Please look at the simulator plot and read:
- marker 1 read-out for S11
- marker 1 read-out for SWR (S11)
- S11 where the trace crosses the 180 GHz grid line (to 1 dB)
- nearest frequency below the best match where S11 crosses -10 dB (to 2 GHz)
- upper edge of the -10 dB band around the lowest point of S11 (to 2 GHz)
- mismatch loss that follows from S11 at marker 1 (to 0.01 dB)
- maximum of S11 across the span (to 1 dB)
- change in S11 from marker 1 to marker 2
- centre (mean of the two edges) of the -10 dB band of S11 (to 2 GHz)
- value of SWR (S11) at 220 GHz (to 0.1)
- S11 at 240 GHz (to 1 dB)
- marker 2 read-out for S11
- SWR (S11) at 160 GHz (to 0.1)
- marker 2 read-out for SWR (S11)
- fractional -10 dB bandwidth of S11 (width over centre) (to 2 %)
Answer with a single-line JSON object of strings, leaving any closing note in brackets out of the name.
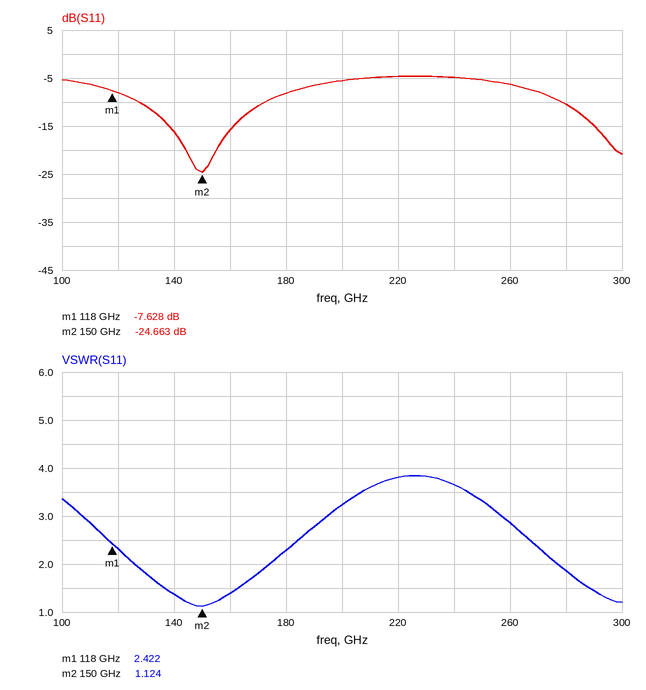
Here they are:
{"marker 1 read-out for S11": "-7.628 dB", "marker 1 read-out for SWR": "2.422", "S11 where the trace crosses the 180 GHz grid line": "-8 dB", "nearest frequency below the best match where S11 crosses -10 dB": "128 GHz", "upper edge of the -10 dB band around the lowest point of S11": "172 GHz", "mismatch loss that follows from S11 at marker 1": "0.82 dB", "maximum of S11 across the span": "-5 dB", "change in S11 from marker 1 to marker 2": "-17.035 dB", "centre (mean of the two edges) of the -10 dB band of S11": "150 GHz", "value of SWR (S11) at 220 GHz": "3.8", "S11 at 240 GHz": "-5 dB", "marker 2 read-out for S11": "-24.663 dB", "SWR (S11) at 160 GHz": "1.4", "marker 2 read-out for SWR": "1.124", "fractional -10 dB bandwidth of S11 (width over centre)": "30 %"}
